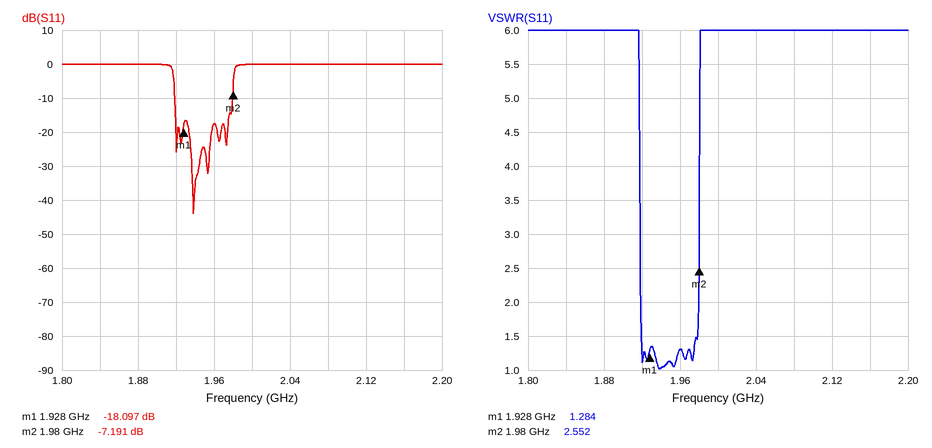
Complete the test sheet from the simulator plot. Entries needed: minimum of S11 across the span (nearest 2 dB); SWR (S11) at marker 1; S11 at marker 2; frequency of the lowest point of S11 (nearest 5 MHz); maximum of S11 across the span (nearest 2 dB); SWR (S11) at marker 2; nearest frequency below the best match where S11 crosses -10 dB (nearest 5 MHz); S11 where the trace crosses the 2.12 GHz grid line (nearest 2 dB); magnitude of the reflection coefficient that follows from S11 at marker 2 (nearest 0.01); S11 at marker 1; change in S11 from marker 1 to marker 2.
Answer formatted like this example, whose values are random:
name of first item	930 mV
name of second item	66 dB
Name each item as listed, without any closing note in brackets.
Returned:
minimum of S11 across the span	-44 dB
SWR (S11) at marker 1	1.284
S11 at marker 2	-7.191 dB
frequency of the lowest point of S11	1.940 GHz
maximum of S11 across the span	0 dB
SWR (S11) at marker 2	2.552
nearest frequency below the best match where S11 crosses -10 dB	1.920 GHz
S11 where the trace crosses the 2.12 GHz grid line	0 dB
magnitude of the reflection coefficient that follows from S11 at marker 2	0.44
S11 at marker 1	-18.097 dB
change in S11 from marker 1 to marker 2	10.906 dB
